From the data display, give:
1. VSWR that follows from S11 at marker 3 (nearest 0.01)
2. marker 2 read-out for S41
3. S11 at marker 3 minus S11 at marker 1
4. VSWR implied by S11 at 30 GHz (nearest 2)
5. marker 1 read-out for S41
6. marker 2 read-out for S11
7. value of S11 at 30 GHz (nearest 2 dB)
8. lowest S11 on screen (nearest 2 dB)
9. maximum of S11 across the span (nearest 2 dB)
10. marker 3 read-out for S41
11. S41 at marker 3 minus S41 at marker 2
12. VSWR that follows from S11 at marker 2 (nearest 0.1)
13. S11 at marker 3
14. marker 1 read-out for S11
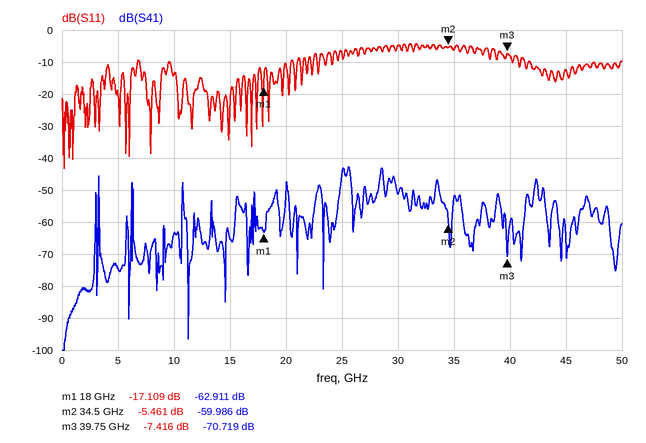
2.48
-59.986 dB
9.693 dB
4
-62.911 dB
-5.461 dB
-4 dB
-44 dB
-4 dB
-70.719 dB
-10.733 dB
3.3
-7.416 dB
-17.109 dB
